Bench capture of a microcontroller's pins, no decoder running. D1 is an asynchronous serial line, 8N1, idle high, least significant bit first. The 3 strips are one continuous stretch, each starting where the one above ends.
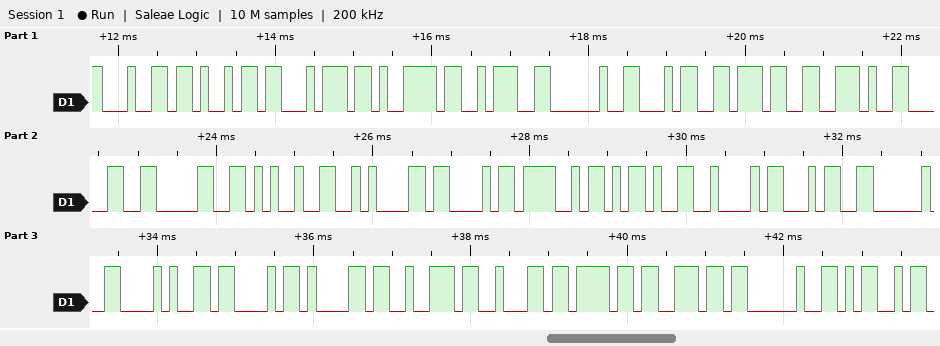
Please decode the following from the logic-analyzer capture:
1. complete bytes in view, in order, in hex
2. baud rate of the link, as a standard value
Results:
0x64 0x69 0x74 0x79 0x3A 0x20 0x34 0x37 0x2E 0x30 0x30 0x25 0x0A 0x43 0x4F 0x2D 0x42 0x34 0x20 0x28 0x43 0x61 0x72 0x62 0x6F 0x6E 0x20 0x4D
9600 baud
